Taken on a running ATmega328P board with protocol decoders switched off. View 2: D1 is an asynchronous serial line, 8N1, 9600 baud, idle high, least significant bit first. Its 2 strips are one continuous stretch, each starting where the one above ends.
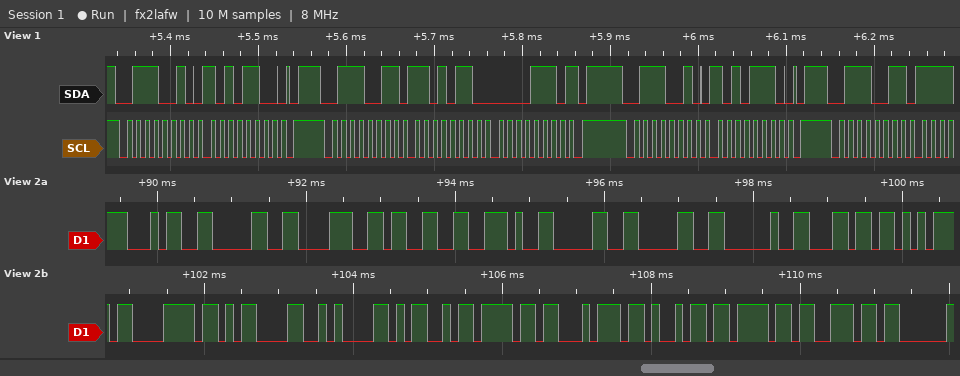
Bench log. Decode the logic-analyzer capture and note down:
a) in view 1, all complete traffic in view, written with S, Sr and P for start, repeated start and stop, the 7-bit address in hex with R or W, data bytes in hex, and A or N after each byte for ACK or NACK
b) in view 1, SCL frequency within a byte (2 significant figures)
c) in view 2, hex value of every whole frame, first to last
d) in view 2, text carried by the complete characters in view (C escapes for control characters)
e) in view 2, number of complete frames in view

S 39W A AC A P S 39R A D6 A 0E N P S 39W A AE A P S 39R A
100 kHz
34 30 38 33 2E 30 30 20 6C 75 78 0D 0A 4D 6F 74 69 6F 6E
"4083.00 lux\r\nMotion"
19
